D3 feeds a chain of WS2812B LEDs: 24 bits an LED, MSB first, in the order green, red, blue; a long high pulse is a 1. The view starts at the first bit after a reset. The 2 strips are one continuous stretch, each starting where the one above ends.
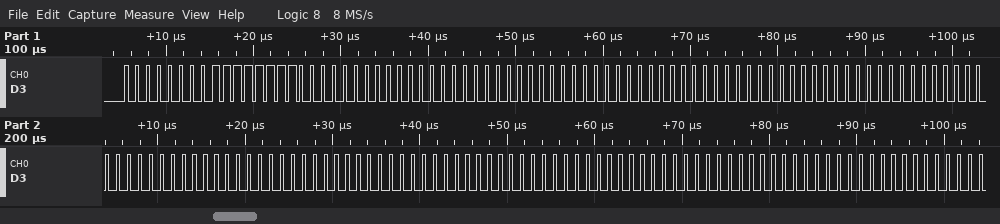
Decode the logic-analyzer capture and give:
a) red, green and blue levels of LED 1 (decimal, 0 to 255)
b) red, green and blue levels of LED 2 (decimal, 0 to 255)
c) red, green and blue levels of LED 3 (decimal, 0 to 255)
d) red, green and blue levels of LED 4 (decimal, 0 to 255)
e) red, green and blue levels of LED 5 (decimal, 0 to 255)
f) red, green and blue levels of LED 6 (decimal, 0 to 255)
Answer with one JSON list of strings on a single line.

["255, 0, 0", "0, 0, 0", "0, 0, 0", "0, 0, 0", "0, 0, 0", "0, 0, 0"]
